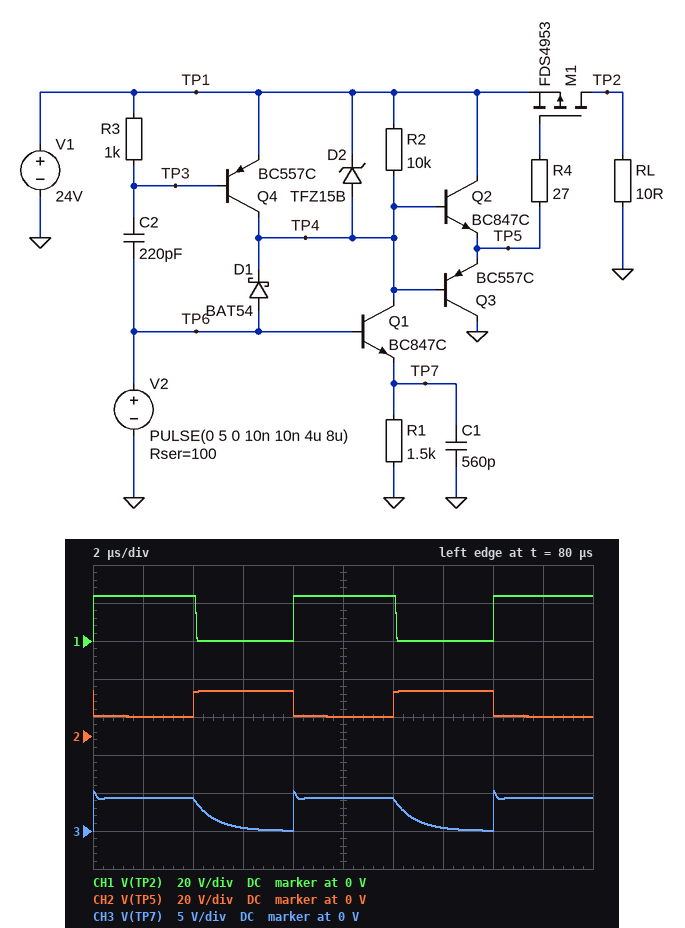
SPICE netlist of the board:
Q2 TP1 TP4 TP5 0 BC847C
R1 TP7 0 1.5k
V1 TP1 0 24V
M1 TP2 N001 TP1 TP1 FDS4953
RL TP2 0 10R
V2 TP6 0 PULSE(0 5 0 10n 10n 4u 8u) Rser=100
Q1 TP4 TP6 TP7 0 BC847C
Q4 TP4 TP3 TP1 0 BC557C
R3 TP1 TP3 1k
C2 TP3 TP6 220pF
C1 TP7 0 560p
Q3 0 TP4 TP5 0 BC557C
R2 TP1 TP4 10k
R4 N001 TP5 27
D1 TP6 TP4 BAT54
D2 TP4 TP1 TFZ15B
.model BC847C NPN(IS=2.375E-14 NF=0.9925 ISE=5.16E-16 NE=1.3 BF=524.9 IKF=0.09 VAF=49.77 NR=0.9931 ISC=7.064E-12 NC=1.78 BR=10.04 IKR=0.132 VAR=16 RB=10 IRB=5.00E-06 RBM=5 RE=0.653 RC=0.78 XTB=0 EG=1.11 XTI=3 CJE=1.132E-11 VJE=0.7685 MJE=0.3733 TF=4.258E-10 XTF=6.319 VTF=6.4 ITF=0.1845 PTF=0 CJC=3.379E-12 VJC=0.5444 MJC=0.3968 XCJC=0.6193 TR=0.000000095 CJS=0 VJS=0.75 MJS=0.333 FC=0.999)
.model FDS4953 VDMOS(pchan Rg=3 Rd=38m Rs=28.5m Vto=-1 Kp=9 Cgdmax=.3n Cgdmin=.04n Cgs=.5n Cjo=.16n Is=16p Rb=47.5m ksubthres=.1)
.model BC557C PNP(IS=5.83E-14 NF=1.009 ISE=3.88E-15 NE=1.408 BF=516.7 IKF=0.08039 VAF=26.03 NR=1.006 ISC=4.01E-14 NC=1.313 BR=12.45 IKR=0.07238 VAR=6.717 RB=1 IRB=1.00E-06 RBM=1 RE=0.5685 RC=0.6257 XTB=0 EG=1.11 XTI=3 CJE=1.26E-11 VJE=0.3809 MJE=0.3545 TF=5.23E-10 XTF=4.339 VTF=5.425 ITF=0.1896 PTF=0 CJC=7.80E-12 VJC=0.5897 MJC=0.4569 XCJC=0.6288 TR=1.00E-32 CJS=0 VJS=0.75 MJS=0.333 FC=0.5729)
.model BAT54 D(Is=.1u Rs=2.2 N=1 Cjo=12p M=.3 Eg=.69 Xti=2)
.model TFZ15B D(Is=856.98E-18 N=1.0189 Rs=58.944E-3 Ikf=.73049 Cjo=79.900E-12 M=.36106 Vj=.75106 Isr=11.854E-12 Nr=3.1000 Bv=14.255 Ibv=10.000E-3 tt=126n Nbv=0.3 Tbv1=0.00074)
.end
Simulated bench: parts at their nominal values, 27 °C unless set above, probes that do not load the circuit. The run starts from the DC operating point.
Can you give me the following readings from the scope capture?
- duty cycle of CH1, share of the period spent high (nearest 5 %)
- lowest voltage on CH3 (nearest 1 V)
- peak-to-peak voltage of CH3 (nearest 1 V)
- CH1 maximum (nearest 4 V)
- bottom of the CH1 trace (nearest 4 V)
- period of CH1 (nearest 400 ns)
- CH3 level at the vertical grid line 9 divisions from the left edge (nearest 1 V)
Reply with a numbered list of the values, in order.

1. 50 %
2. 0 V
3. 5 V
4. 24 V
5. 0 V
6. 8.0 µs
7. 4 V
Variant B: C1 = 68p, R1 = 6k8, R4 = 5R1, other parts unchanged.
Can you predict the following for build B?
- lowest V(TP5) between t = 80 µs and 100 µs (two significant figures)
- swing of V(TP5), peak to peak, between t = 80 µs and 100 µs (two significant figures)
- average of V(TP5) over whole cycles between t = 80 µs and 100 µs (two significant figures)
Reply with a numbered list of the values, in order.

1. 18 V
2. 5.5 V
3. 21 V
